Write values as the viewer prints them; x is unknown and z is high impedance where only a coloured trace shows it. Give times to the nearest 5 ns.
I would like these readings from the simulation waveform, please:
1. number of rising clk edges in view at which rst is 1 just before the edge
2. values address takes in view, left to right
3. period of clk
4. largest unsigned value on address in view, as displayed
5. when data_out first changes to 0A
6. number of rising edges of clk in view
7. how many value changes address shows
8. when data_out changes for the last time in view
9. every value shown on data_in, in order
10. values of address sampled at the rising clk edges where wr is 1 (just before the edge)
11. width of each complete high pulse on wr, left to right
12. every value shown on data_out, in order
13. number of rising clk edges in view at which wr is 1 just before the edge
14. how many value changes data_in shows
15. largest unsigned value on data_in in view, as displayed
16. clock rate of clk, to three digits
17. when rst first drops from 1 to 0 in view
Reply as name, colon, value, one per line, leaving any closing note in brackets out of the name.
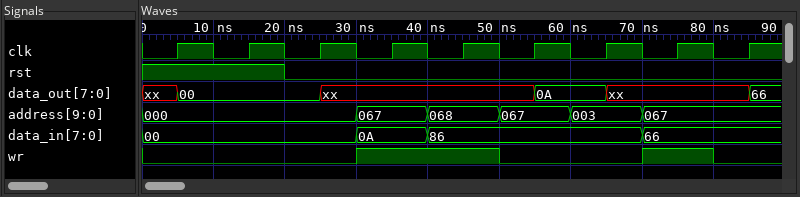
number of rising clk edges in view at which rst is 1 just before the edge: 2
values address takes in view, left to right: 000, 067, 068, 067, 003, 067
period of clk: 10 ns
largest unsigned value on address in view, as displayed: 068
when data_out first changes to 0A: 55 ns
number of rising edges of clk in view: 9
how many value changes address shows: 5
when data_out changes for the last time in view: 85 ns
every value shown on data_in, in order: 00, 0A, 86, 66
values of address sampled at the rising clk edges where wr is 1: 067, 068, 067
width of each complete high pulse on wr, left to right: 20 ns, 10 ns
every value shown on data_out, in order: xx, 00, xx, 0A, xx, 66
number of rising clk edges in view at which wr is 1 just before the edge: 3
how many value changes data_in shows: 3
largest unsigned value on data_in in view, as displayed: 86
clock rate of clk, to three digits: 100 MHz
when rst first drops from 1 to 0 in view: 20 ns
